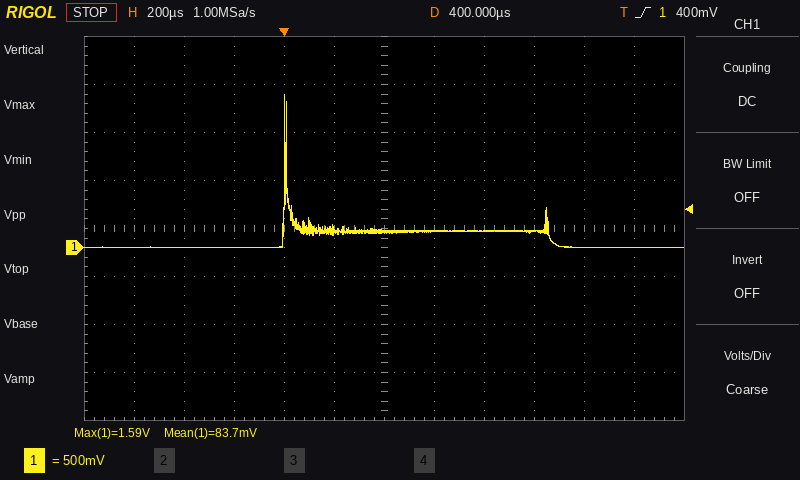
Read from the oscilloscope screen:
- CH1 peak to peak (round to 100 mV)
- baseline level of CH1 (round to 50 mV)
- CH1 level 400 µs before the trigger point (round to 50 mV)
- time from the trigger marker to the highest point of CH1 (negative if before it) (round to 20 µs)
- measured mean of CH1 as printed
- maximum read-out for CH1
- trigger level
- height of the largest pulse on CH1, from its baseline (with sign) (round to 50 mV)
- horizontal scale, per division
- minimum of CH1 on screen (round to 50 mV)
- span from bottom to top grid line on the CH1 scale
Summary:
1.60 V
0 mV
0 mV
0 µs
83.7 mV
1.59 V
400 mV
+1.60 V
200 µs
0 mV
4 V
